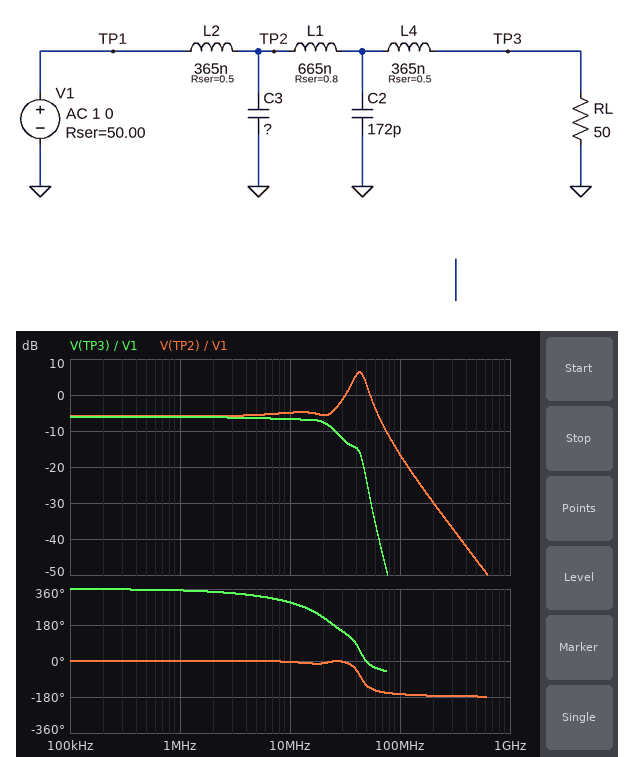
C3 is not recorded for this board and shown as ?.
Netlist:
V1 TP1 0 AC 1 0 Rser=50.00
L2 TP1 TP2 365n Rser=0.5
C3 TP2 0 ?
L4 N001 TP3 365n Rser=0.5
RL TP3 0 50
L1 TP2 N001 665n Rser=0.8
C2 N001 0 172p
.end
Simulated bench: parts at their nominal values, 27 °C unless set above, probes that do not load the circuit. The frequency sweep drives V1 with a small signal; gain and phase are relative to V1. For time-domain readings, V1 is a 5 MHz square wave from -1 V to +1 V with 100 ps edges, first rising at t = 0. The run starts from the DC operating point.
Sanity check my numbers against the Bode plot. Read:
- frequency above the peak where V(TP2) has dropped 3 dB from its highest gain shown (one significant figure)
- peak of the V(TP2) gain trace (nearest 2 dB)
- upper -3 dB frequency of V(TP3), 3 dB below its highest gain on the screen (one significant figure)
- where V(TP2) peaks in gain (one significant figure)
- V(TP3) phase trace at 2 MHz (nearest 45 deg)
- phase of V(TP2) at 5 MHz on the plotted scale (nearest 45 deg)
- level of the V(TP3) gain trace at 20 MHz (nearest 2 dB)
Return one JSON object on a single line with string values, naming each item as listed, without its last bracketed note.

{"frequency above the peak where V(TP2) has dropped 3 dB from its highest gain shown": "50 MHz", "peak of the V(TP2) gain trace": "6 dB", "upper -3 dB frequency of V(TP3), 3 dB below its highest gain on the screen": "20 MHz", "where V(TP2) peaks in gain": "40 MHz", "V(TP3) phase trace at 2 MHz": "360 deg", "phase of V(TP2) at 5 MHz on the plotted scale": "0 deg", "level of the V(TP3) gain trace at 20 MHz": "-8 dB"}
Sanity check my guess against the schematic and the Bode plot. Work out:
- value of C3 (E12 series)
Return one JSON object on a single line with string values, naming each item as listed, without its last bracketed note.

{"value of C3": "56 pF"}
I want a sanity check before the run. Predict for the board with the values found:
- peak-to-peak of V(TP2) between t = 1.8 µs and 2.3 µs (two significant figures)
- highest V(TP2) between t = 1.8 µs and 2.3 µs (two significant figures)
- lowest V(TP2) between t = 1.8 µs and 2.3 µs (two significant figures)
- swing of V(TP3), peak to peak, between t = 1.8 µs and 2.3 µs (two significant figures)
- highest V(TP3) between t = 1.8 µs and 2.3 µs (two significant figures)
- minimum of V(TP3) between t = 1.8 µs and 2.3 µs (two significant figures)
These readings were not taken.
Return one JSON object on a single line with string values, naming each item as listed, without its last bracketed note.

{"peak-to-peak of V(TP2) between t = 1.8 µs and 2.3 µs": "2.4 V", "highest V(TP2) between t = 1.8 µs and 2.3 µs": "1.2 V", "lowest V(TP2) between t = 1.8 µs and 2.3 µs": "-1.2 V", "swing of V(TP3), peak to peak, between t = 1.8 µs and 2.3 µs": "1.0 V", "highest V(TP3) between t = 1.8 µs and 2.3 µs": "510 mV", "minimum of V(TP3) between t = 1.8 µs and 2.3 µs": "-510 mV"}
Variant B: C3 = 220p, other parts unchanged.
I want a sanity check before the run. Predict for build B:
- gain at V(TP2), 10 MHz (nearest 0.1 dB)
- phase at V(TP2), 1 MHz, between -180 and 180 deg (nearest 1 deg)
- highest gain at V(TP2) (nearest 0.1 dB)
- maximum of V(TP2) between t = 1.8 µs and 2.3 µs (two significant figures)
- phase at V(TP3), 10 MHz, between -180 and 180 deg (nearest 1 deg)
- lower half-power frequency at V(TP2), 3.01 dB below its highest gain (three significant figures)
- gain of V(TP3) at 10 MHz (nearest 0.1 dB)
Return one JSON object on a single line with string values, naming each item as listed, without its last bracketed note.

{"gain at V(TP2), 10 MHz": "-4.4 dB", "phase at V(TP2), 1 MHz, between -180 and 180 deg": "-1 deg", "highest gain at V(TP2)": "-2.7 dB", "maximum of V(TP2) between t = 1.8 µs and 2.3 µs": "800 mV", "phase at V(TP3), 10 MHz, between -180 and 180 deg": "-86 deg", "lower half-power frequency at V(TP2), 3.01 dB below its highest gain": "3.05 MHz", "gain of V(TP3) at 10 MHz": "-6.2 dB"}
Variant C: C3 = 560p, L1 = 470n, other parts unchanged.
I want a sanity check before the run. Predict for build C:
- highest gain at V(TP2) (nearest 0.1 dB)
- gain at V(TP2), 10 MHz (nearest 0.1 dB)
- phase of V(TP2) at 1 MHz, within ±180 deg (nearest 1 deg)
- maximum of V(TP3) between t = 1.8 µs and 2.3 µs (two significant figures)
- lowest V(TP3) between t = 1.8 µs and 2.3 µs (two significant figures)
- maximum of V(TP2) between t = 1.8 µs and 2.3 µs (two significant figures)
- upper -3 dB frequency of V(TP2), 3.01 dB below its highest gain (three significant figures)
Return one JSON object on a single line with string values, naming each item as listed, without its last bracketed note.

{"highest gain at V(TP2)": "-5.8 dB", "gain at V(TP2), 10 MHz": "-6.8 dB", "phase of V(TP2) at 1 MHz, within ±180 deg": "-5 deg", "maximum of V(TP3) between t = 1.8 µs and 2.3 µs": "530 mV", "lowest V(TP3) between t = 1.8 µs and 2.3 µs": "-530 mV", "maximum of V(TP2) between t = 1.8 µs and 2.3 µs": "570 mV", "upper -3 dB frequency of V(TP2), 3.01 dB below its highest gain": "13.8 MHz"}
